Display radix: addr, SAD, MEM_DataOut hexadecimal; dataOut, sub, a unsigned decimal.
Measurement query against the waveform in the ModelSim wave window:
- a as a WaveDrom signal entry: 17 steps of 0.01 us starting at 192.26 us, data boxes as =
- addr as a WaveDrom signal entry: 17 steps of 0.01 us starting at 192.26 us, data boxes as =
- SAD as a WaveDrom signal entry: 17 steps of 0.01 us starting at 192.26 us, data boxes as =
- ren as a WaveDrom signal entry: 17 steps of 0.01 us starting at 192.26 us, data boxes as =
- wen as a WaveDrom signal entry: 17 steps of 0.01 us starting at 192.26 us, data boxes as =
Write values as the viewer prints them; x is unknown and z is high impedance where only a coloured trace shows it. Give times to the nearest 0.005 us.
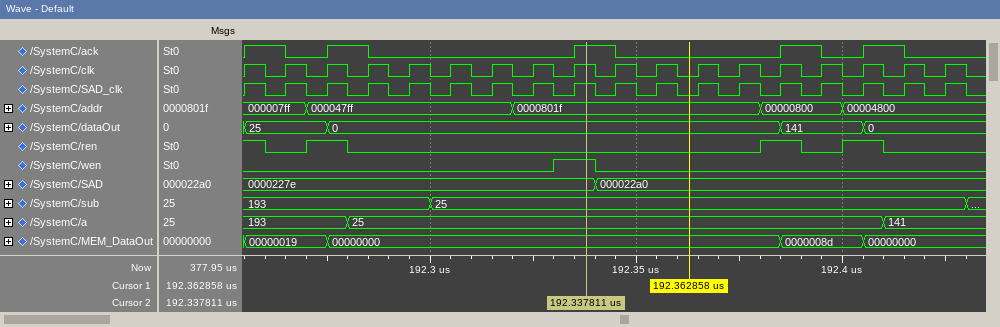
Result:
{name: 'a', wave: '=.=............=.', data: '193 25 141'}
{name: 'addr', wave: '==....=.....=.=..', data: '000007ff 000047ff 0000801f 00000800 00004800'}
{name: 'SAD', wave: '=.......=........', data: '0000227e 000022a0'}
{name: 'ren', wave: '010.........1010.'}
{name: 'wen', wave: '0......10........'}
